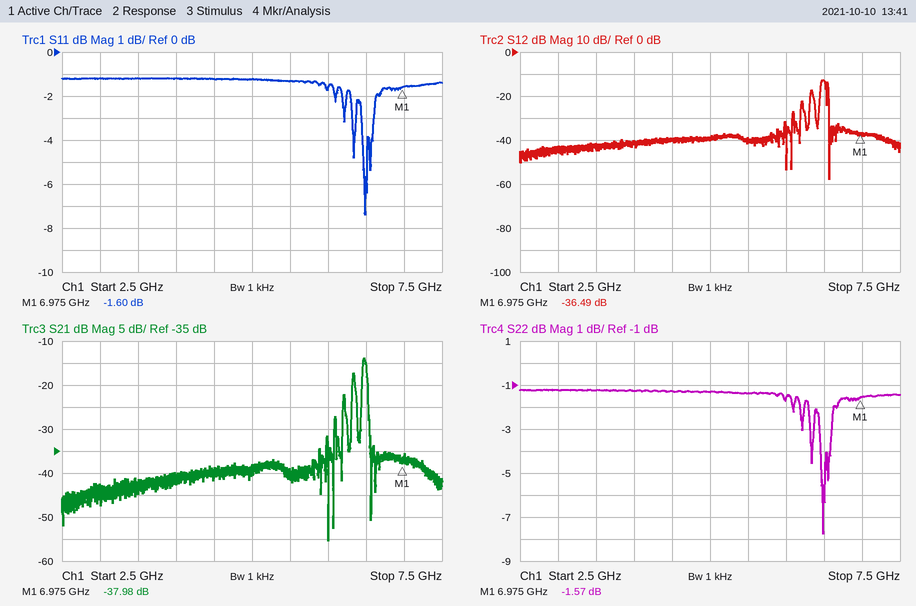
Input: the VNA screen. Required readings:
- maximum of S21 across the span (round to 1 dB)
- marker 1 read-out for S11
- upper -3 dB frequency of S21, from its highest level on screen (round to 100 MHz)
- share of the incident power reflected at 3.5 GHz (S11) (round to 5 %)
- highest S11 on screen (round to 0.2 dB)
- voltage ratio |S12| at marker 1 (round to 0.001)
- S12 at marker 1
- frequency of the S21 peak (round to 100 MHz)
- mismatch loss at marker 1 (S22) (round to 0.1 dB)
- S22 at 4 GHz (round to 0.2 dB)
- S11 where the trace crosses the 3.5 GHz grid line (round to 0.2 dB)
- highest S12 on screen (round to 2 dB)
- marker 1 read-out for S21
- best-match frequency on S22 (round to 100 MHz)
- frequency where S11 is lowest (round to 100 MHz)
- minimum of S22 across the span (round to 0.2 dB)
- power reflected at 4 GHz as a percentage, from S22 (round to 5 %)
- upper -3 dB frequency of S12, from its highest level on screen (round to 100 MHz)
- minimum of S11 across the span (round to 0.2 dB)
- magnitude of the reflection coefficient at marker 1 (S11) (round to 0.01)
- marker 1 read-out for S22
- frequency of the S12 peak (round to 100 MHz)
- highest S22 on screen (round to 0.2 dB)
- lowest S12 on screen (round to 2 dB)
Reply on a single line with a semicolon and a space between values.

-14 dB; -1.60 dB; 6.5 GHz; 75 %; -1.2 dB; 0.015; -36.49 dB; 6.5 GHz; 5.2 dB; -1.2 dB; -1.2 dB; -12 dB; -37.98 dB; 6.5 GHz; 6.5 GHz; -7.8 dB; 75 %; 6.5 GHz; -7.4 dB; 0.83; -1.57 dB; 6.5 GHz; -1.2 dB; -58 dB
